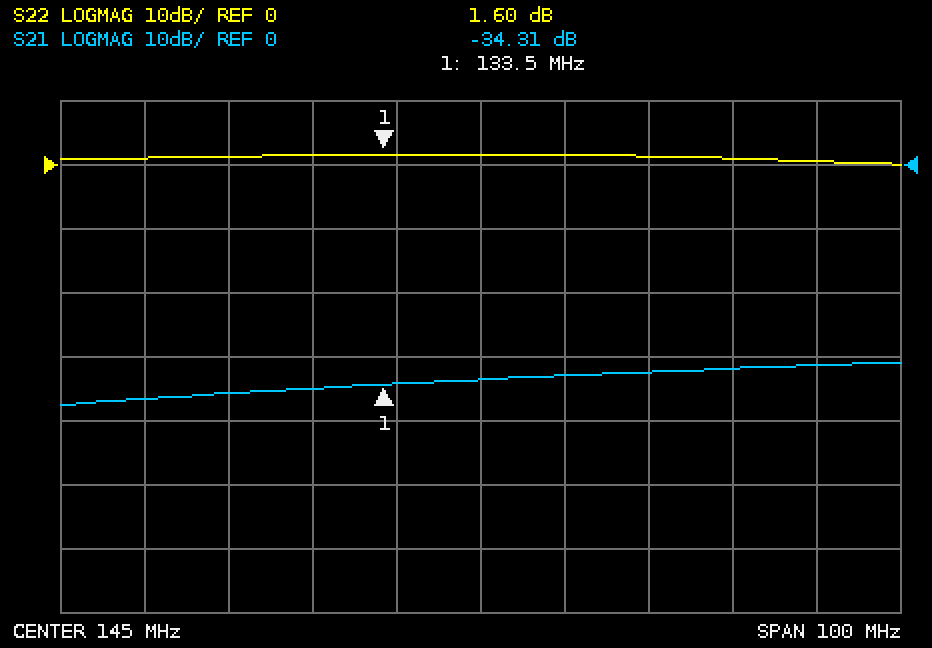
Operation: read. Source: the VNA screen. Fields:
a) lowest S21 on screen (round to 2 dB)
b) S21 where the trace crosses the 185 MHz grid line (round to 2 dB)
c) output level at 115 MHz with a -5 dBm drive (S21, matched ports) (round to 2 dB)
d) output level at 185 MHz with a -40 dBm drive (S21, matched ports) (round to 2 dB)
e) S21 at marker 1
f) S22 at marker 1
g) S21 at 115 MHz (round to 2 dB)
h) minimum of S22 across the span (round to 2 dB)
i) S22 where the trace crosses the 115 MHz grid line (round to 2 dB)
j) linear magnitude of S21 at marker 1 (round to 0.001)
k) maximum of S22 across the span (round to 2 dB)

-38 dB
-32 dB
-40 dBm
-72 dBm
-34.31 dB
1.60 dB
-36 dB
0 dB
2 dB
0.019
2 dB
